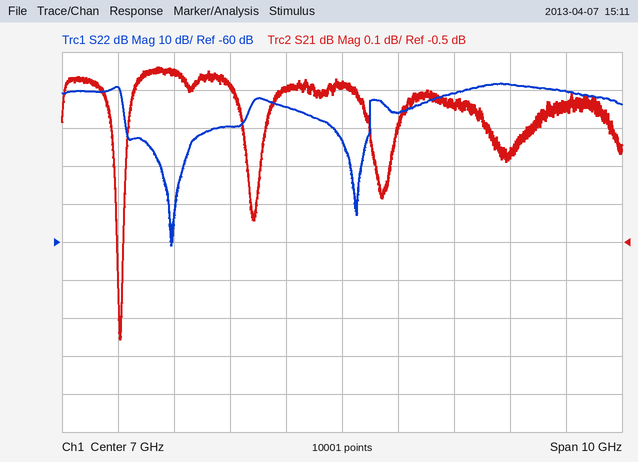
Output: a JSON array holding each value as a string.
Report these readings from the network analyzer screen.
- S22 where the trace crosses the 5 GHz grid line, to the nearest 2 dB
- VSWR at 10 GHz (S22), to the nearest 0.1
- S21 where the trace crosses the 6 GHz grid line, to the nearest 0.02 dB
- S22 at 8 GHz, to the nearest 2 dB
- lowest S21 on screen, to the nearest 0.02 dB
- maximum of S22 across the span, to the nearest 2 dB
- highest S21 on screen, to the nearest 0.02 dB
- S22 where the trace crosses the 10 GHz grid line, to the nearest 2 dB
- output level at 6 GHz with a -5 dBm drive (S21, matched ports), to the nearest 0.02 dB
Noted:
["-30 dB", "1.3", "-0.10 dB", "-26 dB", "-0.76 dB", "-18 dB", "-0.04 dB", "-18 dB", "-5.10 dBm"]
